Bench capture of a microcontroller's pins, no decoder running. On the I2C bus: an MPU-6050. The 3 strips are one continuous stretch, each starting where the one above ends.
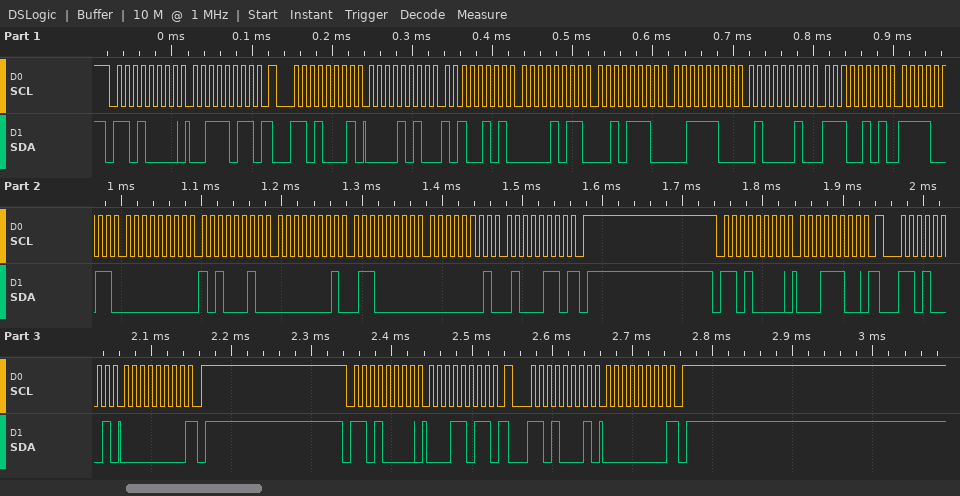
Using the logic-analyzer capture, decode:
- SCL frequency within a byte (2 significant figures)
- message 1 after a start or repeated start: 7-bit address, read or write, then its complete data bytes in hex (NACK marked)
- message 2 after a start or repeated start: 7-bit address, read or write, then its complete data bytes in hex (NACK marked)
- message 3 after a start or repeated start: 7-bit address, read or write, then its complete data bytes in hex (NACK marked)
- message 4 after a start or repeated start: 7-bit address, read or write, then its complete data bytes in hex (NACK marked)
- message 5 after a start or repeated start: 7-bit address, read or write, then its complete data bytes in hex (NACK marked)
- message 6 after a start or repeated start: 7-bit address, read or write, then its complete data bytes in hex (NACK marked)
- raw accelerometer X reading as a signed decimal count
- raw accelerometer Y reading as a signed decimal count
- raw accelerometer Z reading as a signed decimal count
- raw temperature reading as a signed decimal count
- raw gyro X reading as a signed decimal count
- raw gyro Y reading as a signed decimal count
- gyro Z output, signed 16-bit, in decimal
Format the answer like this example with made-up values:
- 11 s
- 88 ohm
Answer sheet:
- 100 kHz
- 0x68 write: 3B
- 0x68 read: 0A A5 0B 2E 3C 42 E5 F3 00 A2 01 60 01 46 NACK
- 0x68 write: 1C
- 0x68 read: 00 NACK
- 0x68 write: 1B
- 0x68 read: 00 NACK
- 2725
- 2862
- 15426
- -6669
- 162
- 352
- 326
